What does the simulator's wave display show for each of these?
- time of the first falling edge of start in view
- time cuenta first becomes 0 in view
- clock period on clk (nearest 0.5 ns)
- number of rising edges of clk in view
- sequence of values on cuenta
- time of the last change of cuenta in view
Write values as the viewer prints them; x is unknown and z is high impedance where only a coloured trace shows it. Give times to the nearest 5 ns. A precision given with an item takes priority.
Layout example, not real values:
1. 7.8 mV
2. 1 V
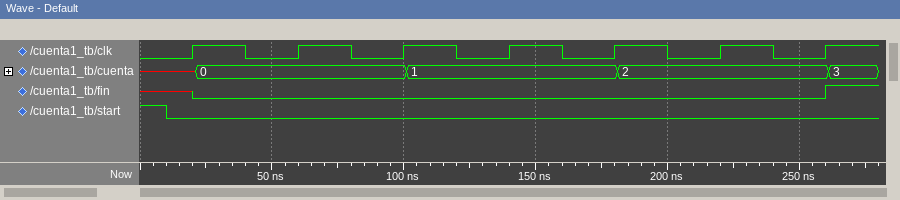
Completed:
1. 10 ns
2. 20 ns
3. 40 ns
4. 7
5. x, 0, 1, 2, 3
6. 260 ns
